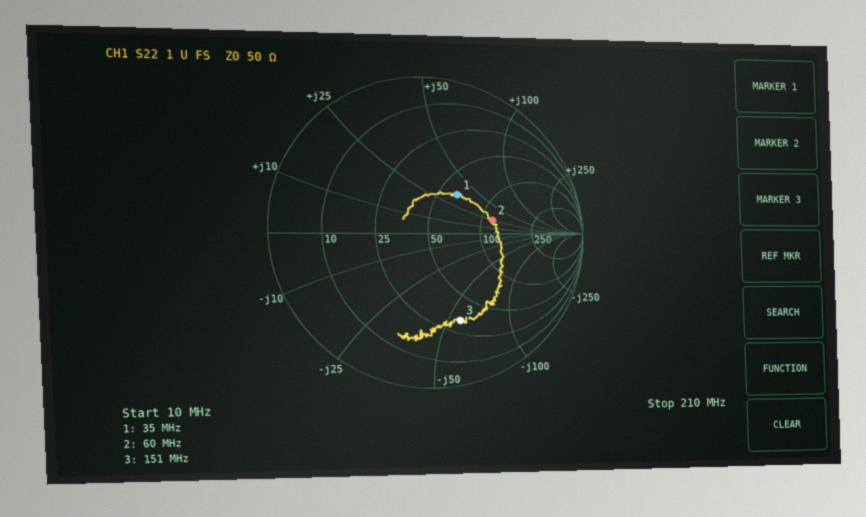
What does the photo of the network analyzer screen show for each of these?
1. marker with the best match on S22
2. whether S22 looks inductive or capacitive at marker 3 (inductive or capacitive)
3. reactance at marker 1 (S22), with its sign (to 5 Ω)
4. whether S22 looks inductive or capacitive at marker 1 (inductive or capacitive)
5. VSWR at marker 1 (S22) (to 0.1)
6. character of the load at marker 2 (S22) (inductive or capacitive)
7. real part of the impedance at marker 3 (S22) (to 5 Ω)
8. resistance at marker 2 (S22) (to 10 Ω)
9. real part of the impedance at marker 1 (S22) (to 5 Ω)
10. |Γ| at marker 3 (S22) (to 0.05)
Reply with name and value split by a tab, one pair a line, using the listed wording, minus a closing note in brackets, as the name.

marker with the best match on S22	marker 1
whether S22 looks inductive or capacitive at marker 3	capacitive
reactance at marker 1 (S22), with its sign	+35 Ω
whether S22 looks inductive or capacitive at marker 1	inductive
VSWR at marker 1 (S22)	1.9
character of the load at marker 2 (S22)	inductive
real part of the impedance at marker 3 (S22)	35 Ω
resistance at marker 2 (S22)	120 Ω
real part of the impedance at marker 1 (S22)	65 Ω
|Γ| at marker 3 (S22)	0.60
